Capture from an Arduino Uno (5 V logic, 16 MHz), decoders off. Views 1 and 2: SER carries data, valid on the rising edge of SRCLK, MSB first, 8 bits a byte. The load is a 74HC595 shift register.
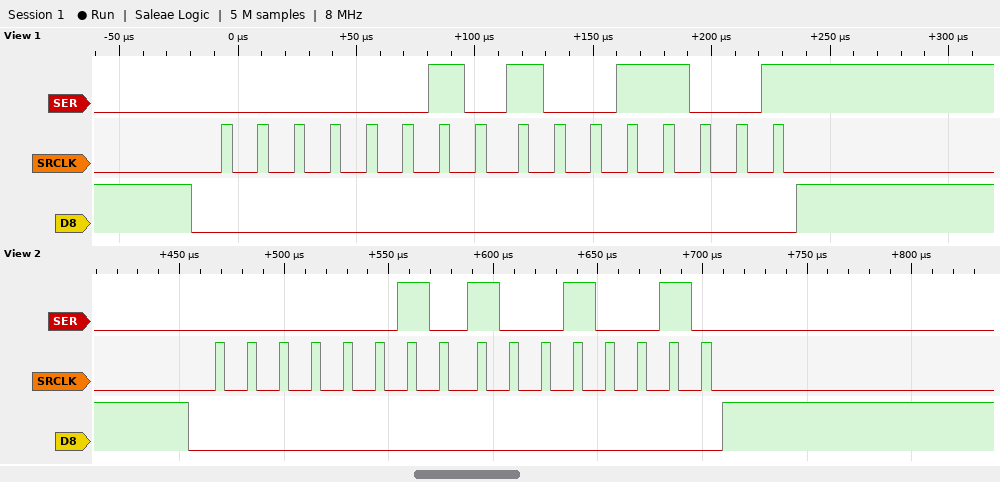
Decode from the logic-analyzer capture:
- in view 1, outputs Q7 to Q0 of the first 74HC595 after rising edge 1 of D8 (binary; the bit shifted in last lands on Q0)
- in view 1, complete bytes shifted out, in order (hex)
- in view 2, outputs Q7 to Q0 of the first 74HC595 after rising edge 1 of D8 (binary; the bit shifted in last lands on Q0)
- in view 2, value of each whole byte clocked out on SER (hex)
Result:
10011001
02 99
10010010
02 92
